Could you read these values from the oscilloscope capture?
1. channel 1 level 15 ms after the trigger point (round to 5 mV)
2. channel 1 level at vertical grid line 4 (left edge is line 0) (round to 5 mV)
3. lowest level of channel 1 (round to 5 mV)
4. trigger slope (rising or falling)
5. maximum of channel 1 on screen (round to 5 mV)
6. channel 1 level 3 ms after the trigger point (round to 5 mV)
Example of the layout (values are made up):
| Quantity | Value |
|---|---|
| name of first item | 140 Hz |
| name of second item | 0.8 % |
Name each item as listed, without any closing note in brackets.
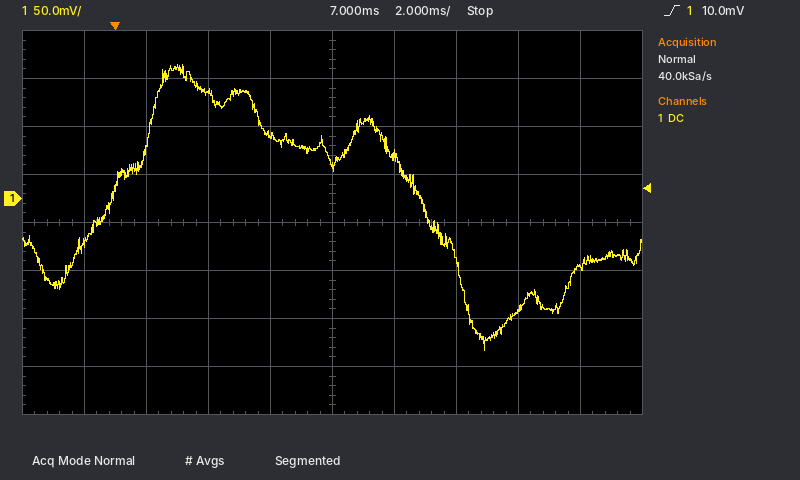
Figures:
| Quantity | Value |
|---|---|
| channel 1 level 15 ms after the trigger point | -70 mV |
| channel 1 level at vertical grid line 4 (left edge is line 0) | 65 mV |
| lowest level of channel 1 | -160 mV |
| trigger slope | rising |
| maximum of channel 1 on screen | 140 mV |
| channel 1 level 3 ms after the trigger point | 110 mV |
